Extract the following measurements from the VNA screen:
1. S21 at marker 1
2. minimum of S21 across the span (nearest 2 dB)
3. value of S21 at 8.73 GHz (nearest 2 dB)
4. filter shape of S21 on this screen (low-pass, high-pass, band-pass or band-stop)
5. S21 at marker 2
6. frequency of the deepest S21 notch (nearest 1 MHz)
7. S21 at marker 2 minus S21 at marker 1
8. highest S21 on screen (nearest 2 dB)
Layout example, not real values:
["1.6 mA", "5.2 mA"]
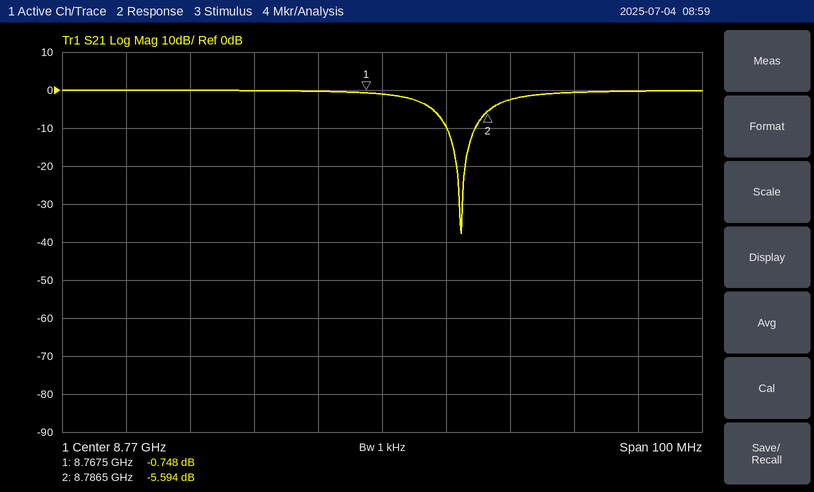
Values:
["-0.748 dB", "-38 dB", "0 dB", "band-stop", "-5.594 dB", "8.782 GHz", "-4.846 dB", "0 dB"]
